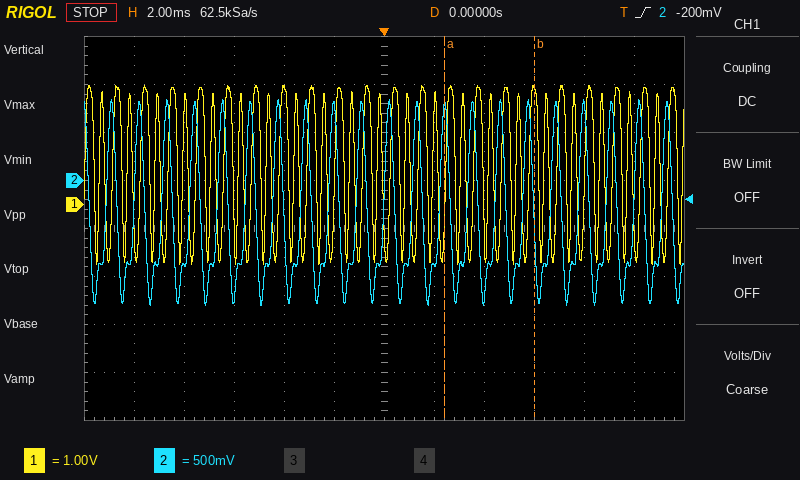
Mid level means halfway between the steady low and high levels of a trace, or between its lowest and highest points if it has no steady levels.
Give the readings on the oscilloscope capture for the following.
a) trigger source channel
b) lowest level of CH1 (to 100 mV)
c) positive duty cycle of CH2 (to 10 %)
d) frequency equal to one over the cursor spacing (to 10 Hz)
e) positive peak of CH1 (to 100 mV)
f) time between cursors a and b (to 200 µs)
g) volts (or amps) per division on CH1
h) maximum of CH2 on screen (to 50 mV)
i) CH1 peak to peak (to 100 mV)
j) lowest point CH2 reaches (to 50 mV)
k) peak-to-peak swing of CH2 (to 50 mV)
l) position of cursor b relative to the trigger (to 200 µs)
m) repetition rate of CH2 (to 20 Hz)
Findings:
CH2
-1.2 V
40 %
280 Hz
2.5 V
3.6 ms
1 V
850 mV
3.7 V
-1.30 V
2.15 V
+6.0 ms
900 Hz
